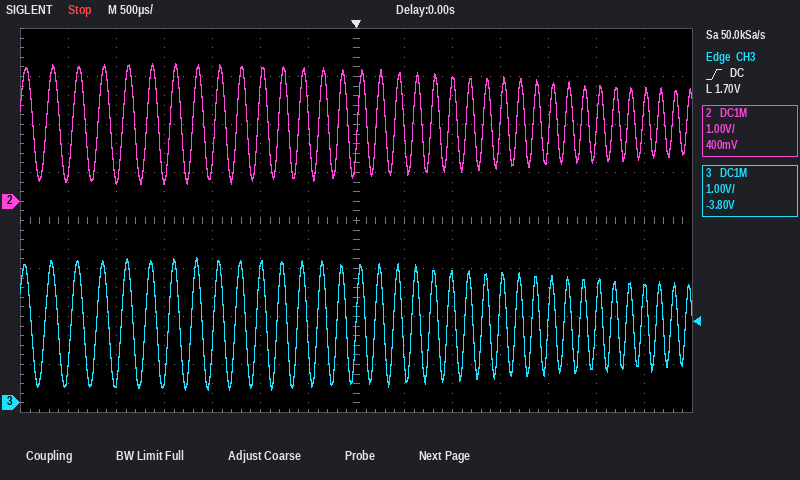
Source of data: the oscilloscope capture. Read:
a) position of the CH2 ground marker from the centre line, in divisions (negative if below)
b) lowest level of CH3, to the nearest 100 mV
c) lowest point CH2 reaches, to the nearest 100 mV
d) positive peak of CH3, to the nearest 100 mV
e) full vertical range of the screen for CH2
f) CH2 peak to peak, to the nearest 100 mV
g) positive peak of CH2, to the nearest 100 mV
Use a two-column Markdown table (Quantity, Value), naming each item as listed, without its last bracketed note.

| Quantity | Value |
|---|---|
| position of the CH2 ground marker from the centre line, in divisions | +0.4 div |
| lowest level of CH3, to the nearest 100 mV | 300 mV |
| lowest point CH2 reaches, to the nearest 100 mV | 400 mV |
| positive peak of CH3, to the nearest 100 mV | 3.0 V |
| full vertical range of the screen for CH2 | 8 V |
| CH2 peak to peak, to the nearest 100 mV | 2.5 V |
| positive peak of CH2, to the nearest 100 mV | 2.9 V |
